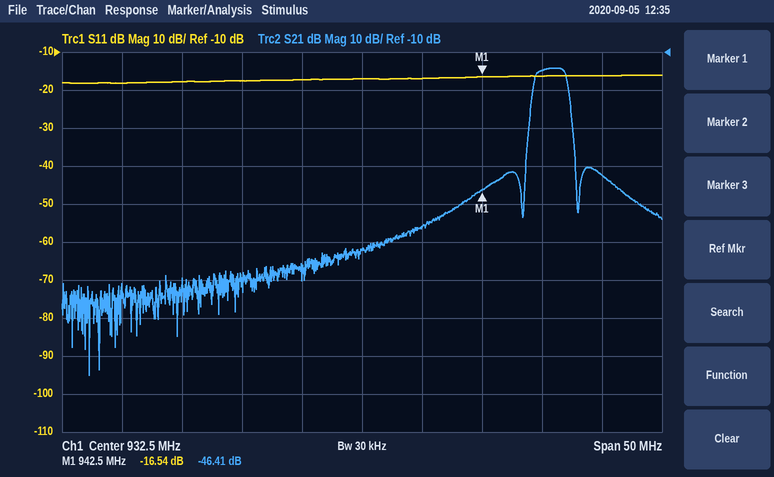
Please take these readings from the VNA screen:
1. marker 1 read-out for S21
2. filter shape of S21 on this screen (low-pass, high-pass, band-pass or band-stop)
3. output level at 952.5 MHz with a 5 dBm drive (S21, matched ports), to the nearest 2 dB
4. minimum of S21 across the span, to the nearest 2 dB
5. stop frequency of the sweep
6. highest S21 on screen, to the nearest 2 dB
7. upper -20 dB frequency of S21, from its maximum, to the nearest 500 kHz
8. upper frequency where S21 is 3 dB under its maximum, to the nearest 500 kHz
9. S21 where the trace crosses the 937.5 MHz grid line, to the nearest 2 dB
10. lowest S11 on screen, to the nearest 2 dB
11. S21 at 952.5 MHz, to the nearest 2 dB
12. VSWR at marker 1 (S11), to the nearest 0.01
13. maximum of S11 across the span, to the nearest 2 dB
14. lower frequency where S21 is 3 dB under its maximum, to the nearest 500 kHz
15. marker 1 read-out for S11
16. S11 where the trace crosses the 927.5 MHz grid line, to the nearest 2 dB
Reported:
-46.41 dB
band-pass
-38 dBm
-96 dB
957.5 MHz
-14 dB
950.0 MHz
949.5 MHz
-56 dB
-18 dB
-42 dB
1.35
-16 dB
947.0 MHz
-16.54 dB
-18 dB
